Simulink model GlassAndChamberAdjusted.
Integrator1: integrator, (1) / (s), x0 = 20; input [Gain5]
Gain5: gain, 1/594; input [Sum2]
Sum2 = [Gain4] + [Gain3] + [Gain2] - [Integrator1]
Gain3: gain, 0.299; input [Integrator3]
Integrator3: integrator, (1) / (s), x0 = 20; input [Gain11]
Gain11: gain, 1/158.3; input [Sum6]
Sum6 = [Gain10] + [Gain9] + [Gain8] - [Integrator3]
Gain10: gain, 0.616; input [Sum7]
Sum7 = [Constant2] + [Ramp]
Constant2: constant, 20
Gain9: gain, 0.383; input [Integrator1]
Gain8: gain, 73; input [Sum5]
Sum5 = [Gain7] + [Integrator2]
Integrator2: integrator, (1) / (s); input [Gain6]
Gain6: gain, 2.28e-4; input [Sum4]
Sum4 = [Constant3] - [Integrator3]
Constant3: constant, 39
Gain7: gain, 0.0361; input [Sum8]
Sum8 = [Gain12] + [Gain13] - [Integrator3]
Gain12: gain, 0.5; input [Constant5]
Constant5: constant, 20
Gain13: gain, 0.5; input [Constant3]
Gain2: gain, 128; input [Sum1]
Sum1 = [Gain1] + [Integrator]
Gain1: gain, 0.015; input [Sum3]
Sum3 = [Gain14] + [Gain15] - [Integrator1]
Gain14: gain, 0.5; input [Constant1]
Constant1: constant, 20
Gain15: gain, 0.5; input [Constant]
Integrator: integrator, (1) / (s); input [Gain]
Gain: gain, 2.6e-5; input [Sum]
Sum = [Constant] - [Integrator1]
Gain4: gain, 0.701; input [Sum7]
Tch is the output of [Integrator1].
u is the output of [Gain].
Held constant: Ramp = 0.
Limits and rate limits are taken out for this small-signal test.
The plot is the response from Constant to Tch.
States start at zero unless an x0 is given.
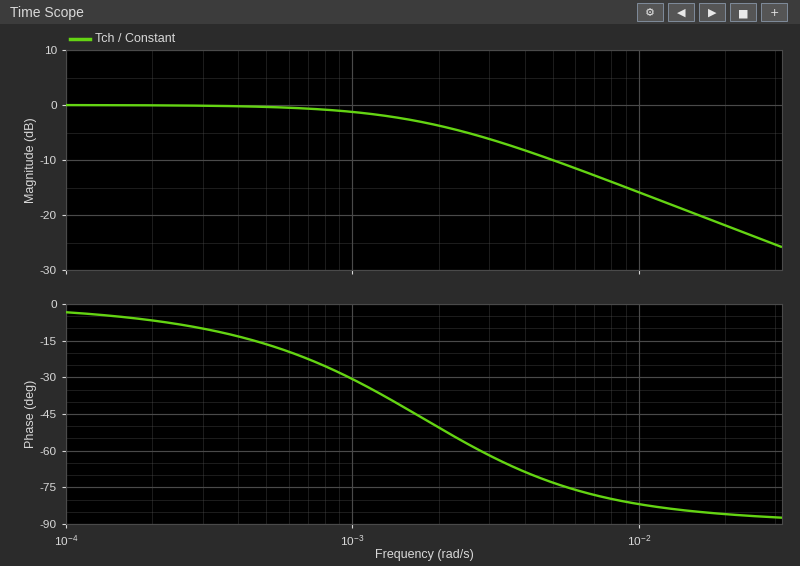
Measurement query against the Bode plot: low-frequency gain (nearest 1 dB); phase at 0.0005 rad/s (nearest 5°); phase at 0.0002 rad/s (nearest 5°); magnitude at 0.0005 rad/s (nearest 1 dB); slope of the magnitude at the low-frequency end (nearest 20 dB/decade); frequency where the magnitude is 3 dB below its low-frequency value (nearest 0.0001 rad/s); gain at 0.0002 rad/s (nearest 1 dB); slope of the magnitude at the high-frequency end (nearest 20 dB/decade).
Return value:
0 dB
-15°
-5°
0 dB
0 dB/decade
0.0017 rad/s
0 dB
-20 dB/decade
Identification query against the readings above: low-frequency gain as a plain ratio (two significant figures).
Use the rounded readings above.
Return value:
1.0
